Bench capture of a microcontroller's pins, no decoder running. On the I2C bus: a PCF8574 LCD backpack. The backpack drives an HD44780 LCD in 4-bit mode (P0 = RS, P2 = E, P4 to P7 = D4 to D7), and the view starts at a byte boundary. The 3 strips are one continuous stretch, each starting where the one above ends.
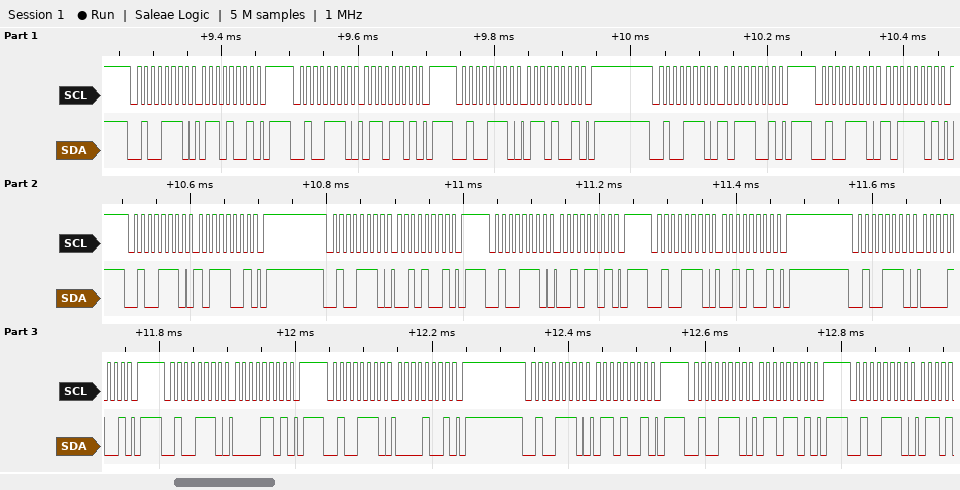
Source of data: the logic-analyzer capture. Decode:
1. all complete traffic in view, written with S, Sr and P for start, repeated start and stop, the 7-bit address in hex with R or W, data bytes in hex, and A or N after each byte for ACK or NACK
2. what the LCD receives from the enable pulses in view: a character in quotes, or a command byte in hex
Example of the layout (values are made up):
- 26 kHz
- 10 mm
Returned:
- S 27W A 69 A P S 27W A 6D A P S 27W A 69 A P S 27W A B9 A P S 27W A BD A P S 27W A B9 A P S 27W A 29 A P S 27W A 2D A P S 27W A 29 A P S 27W A 09 A P S 27W A 0D A P S 27W A 09 A P S 27W A 69 A P S 27W A 6D A P S 27W A
- 'k' ' '
